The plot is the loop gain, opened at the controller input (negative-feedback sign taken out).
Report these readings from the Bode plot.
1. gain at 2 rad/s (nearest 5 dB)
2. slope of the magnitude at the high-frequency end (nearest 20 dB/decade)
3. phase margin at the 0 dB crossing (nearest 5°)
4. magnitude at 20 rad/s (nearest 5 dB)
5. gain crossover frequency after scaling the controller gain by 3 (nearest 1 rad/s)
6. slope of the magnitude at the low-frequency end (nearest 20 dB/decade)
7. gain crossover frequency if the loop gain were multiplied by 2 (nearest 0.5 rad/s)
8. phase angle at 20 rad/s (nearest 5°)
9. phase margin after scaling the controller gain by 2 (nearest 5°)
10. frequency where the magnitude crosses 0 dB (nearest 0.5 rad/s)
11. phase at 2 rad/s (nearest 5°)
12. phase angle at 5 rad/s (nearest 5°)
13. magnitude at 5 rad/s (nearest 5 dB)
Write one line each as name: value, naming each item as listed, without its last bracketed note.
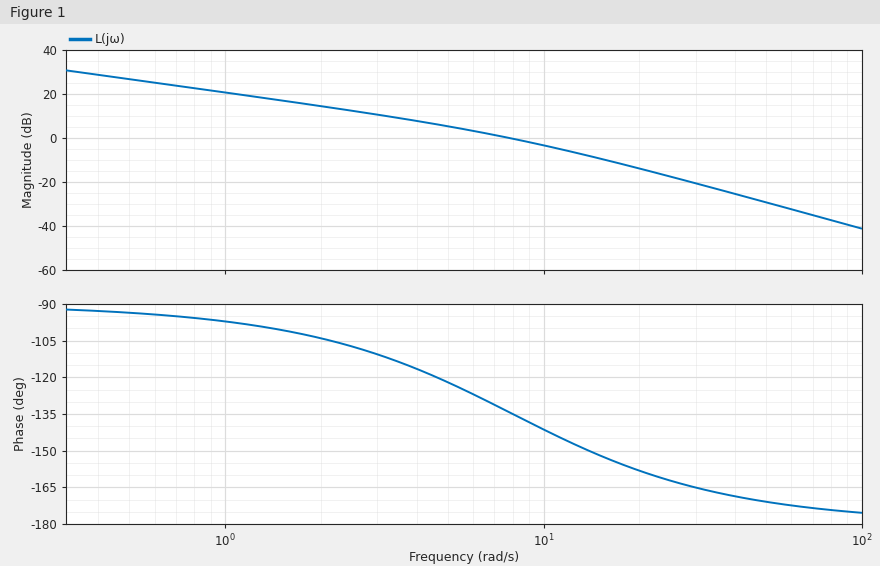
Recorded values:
gain at 2 rad/s: 15 dB
slope of the magnitude at the high-frequency end: -40 dB/decade
phase margin at the 0 dB crossing: 45°
magnitude at 20 rad/s: -15 dB
gain crossover frequency after scaling the controller gain by 3: 15 rad/s
slope of the magnitude at the low-frequency end: -20 dB/decade
gain crossover frequency if the loop gain were multiplied by 2: 12.0 rad/s
phase angle at 20 rad/s: -160°
phase margin after scaling the controller gain by 2: 35°
frequency where the magnitude crosses 0 dB: 8.0 rad/s
phase at 2 rad/s: -105°
phase angle at 5 rad/s: -120°
magnitude at 5 rad/s: 5 dB
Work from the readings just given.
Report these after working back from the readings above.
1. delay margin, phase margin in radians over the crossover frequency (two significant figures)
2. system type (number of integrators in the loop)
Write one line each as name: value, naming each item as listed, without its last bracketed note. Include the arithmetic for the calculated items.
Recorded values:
delay margin, phase margin in radians over the crossover frequency: 45 × π / 180 / 8 = 0.098 s
system type: 1
